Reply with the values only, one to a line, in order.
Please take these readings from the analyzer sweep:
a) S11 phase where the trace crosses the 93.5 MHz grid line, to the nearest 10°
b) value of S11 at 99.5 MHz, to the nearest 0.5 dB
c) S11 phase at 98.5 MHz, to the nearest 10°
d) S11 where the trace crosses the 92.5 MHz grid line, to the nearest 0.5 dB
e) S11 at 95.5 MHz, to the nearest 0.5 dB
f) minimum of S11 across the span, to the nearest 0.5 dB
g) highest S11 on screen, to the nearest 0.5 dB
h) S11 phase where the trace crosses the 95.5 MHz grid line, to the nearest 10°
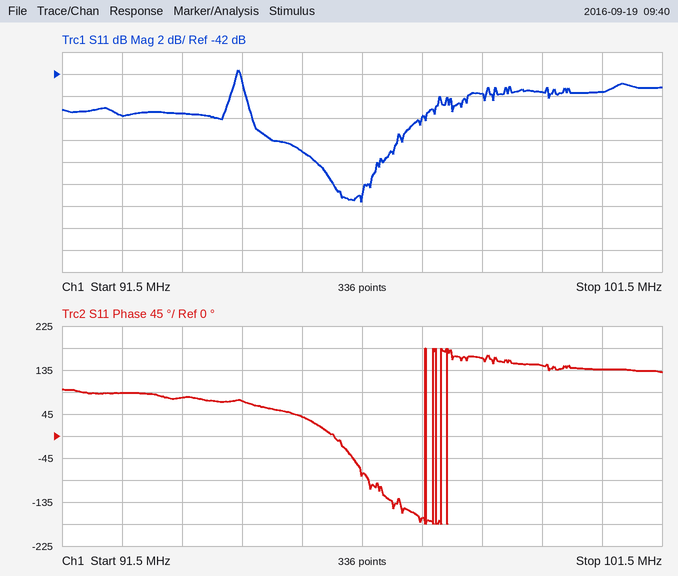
80°
-43.5 dB
160°
-46.0 dB
-49.0 dB
-53.5 dB
-41.5 dB
40°
